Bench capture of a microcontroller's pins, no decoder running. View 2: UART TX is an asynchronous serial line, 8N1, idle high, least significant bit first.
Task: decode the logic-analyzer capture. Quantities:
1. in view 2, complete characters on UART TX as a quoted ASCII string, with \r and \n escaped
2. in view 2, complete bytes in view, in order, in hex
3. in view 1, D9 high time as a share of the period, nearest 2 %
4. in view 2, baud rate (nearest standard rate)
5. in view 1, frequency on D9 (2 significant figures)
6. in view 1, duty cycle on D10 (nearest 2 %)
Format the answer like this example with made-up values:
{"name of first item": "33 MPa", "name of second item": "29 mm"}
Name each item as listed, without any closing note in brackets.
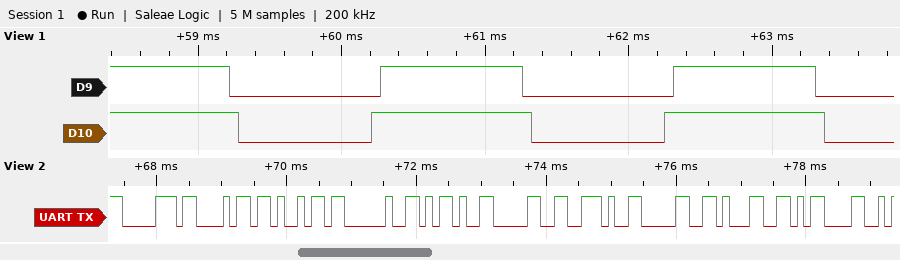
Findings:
{"in view 2, complete characters on UART TX as a quoted ASCII string, with \\r and \\n escaped": "\"phi -0.01\\r\"", "in view 2, complete bytes in view, in order, in hex": "70 68 69 20 2D 30 2E 30 31 0D", "in view 1, D9 high time as a share of the period, nearest 2 %": "48 %", "in view 2, baud rate": "9600 baud", "in view 1, frequency on D9": "490 Hz", "in view 1, duty cycle on D10": "54 %"}
